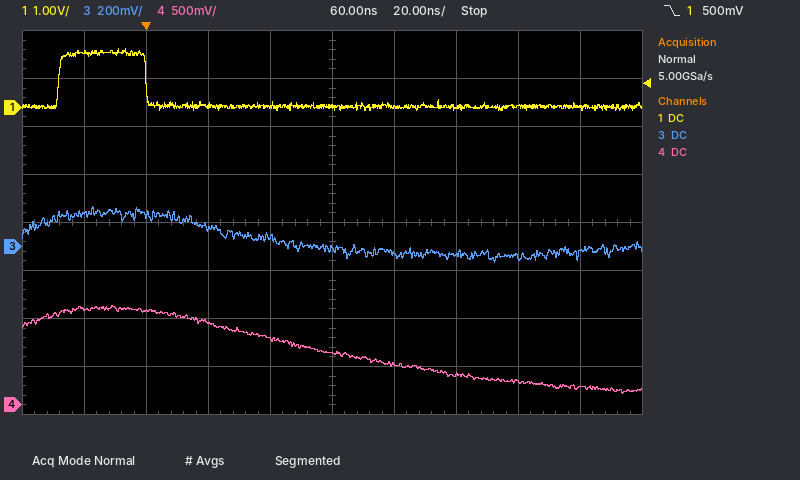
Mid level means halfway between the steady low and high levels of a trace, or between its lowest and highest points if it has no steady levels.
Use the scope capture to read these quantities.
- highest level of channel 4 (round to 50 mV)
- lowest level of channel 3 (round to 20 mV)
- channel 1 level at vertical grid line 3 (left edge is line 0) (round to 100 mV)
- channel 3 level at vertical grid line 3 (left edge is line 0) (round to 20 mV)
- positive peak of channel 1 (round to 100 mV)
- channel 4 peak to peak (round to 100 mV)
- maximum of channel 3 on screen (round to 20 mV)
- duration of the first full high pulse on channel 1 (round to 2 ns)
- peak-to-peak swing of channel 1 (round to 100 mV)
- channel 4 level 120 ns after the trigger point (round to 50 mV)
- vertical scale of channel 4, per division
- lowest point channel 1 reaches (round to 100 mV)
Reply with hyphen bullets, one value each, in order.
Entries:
- 1.05 V
- -60 mV
- 0.0 V
- 80 mV
- 1.2 V
- 900 mV
- 160 mV
- 28 ns
- 1.3 V
- 250 mV
- 500 mV
- -100 mV
